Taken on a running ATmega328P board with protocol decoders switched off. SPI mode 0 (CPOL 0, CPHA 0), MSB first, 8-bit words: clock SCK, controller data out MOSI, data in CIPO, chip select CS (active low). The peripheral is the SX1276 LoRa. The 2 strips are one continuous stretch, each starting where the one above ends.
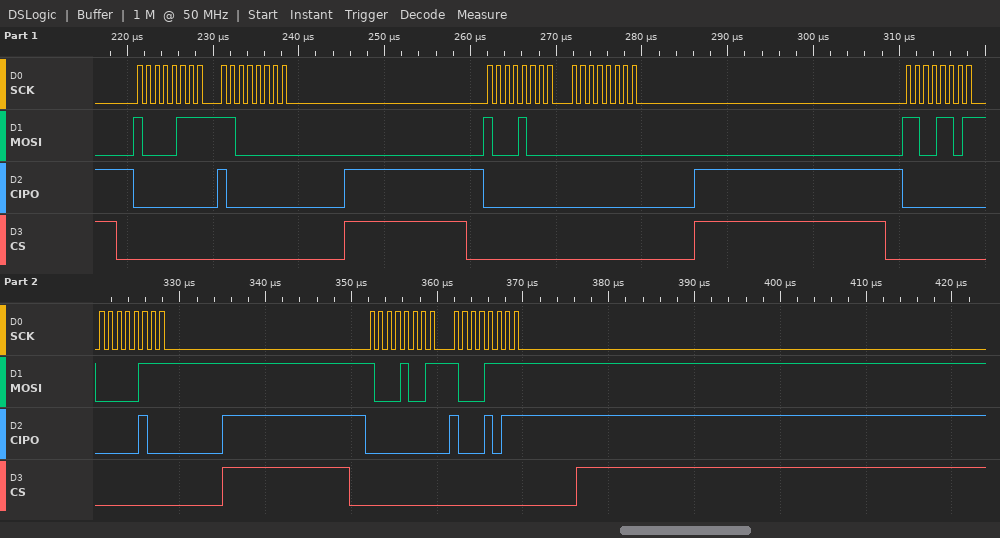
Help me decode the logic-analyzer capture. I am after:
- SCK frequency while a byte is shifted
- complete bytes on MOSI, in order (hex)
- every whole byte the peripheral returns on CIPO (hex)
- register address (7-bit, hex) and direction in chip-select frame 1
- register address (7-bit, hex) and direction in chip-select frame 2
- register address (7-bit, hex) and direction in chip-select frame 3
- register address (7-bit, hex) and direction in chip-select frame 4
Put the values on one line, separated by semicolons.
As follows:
1 MHz; 87 C0 88 00 CD 07 89 8F; 00 80 00 00 00 04 00 8B; 0x07 write; 0x08 write; 0x4D write; 0x09 write
